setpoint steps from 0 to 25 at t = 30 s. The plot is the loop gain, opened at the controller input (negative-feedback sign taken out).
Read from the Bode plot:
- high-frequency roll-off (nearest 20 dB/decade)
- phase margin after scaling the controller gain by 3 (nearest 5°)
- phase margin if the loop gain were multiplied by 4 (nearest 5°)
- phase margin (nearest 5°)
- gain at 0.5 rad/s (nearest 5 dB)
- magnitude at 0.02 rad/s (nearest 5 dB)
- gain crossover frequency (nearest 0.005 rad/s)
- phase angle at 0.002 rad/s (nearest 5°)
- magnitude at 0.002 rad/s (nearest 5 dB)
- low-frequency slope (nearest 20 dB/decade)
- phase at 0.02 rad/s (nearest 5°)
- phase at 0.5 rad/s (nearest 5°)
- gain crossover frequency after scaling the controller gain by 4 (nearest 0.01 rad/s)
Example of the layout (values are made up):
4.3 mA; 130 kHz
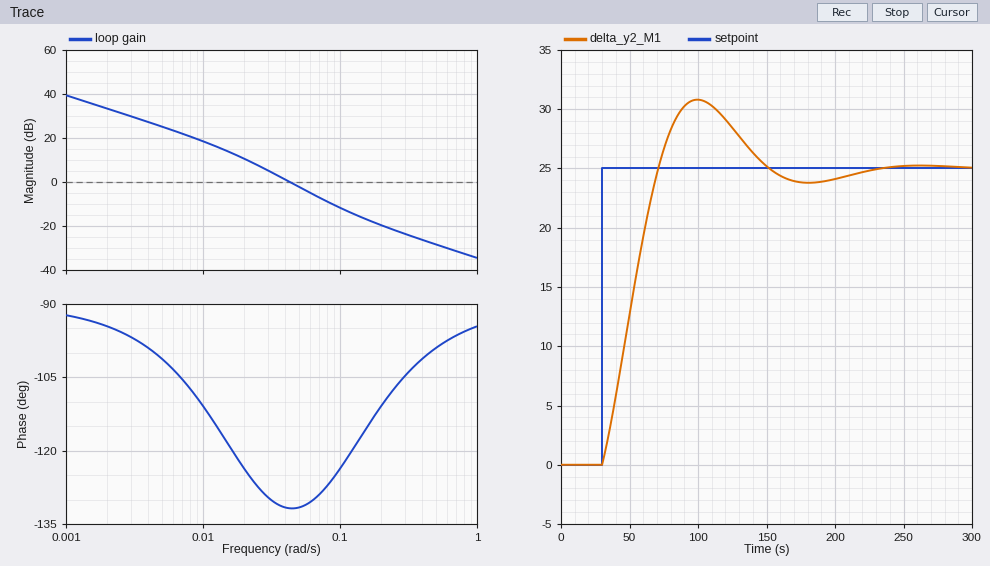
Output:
-20 dB/decade; 55°; 55°; 50°; -30 dB; 10 dB; 0.045 rad/s; -95°; 35 dB; -20 dB/decade; -125°; -100°; 0.10 rad/s
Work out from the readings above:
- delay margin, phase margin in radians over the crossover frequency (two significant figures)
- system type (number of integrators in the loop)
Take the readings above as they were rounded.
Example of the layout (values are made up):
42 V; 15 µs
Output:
19 s; 1
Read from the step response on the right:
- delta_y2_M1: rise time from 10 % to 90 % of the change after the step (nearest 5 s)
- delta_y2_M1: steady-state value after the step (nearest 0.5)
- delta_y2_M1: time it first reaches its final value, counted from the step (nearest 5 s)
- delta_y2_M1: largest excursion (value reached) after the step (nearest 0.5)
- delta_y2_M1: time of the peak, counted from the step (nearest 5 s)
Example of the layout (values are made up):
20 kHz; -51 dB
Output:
30 s; 25.0; 40 s; 31.0; 70 s
